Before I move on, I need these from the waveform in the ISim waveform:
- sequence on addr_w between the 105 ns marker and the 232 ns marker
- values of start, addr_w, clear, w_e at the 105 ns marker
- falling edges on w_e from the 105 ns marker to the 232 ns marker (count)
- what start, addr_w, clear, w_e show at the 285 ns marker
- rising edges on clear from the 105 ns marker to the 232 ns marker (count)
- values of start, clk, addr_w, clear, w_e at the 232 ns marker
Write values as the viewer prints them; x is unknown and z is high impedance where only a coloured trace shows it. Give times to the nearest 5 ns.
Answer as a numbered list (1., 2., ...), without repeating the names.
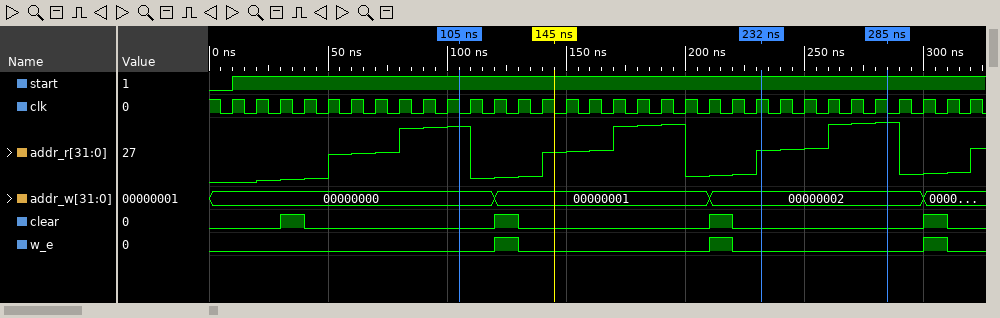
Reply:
1. 00000000, 00000001, 00000002
2. start=1, addr_w=00000000, clear=0, w_e=0
3. 2
4. start=1, addr_w=00000002, clear=0, w_e=0
5. 2
6. start=1, clk=1, addr_w=00000002, clear=0, w_e=0
